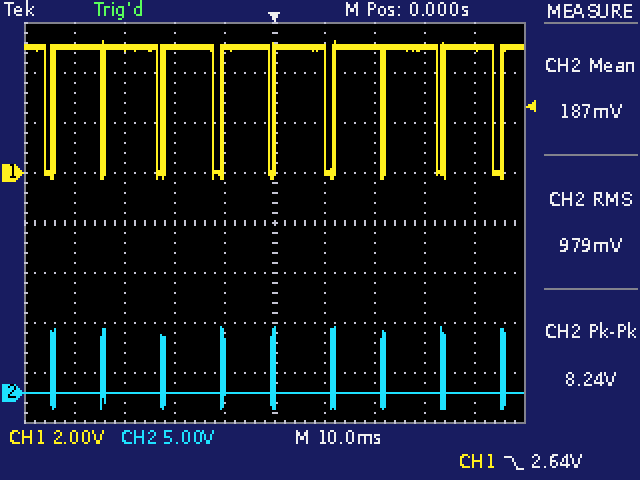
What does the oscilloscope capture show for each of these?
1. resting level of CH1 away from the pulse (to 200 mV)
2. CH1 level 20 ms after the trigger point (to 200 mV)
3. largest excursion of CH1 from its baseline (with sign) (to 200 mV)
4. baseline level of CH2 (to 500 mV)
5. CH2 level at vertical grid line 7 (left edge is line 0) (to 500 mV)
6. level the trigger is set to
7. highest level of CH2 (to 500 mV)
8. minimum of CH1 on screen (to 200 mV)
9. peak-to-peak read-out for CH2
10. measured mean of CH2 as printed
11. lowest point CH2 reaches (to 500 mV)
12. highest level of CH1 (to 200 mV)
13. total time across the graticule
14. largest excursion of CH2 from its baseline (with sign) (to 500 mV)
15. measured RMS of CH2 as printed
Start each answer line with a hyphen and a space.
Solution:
- 5.0 V
- 5.0 V
- -5.2 V
- 0.0 V
- 0.0 V
- 2.64 V
- 6.5 V
- -200 mV
- 8.24 V
- 187 mV
- -1.5 V
- 5.2 V
- 100 ms
- +6.5 V
- 979 mV
